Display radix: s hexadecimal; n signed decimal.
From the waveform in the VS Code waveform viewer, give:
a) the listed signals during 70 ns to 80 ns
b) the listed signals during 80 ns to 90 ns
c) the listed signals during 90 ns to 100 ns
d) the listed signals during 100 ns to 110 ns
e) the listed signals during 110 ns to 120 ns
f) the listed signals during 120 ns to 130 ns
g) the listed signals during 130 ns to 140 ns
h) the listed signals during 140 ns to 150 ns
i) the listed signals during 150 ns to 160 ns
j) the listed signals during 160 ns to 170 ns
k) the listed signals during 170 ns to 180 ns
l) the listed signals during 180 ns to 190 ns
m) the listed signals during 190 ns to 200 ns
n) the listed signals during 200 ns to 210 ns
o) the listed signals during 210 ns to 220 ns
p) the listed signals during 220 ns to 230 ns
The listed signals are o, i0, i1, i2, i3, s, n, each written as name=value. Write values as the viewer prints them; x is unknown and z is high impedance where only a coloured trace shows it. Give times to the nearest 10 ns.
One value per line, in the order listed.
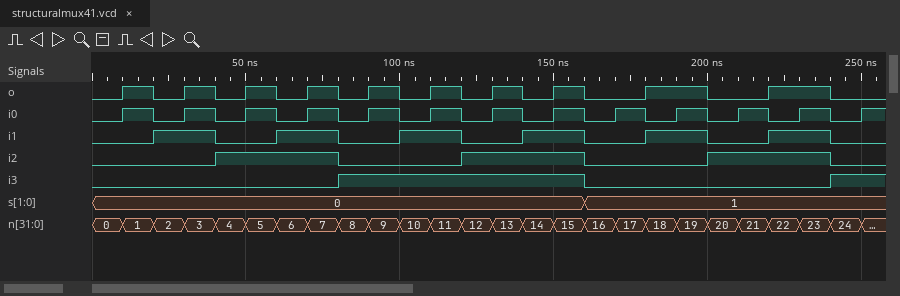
o=1, i0=1, i1=1, i2=1, i3=0, s=0, n=7
o=0, i0=0, i1=0, i2=0, i3=1, s=0, n=8
o=1, i0=1, i1=0, i2=0, i3=1, s=0, n=9
o=0, i0=0, i1=1, i2=0, i3=1, s=0, n=10
o=1, i0=1, i1=1, i2=0, i3=1, s=0, n=11
o=0, i0=0, i1=0, i2=1, i3=1, s=0, n=12
o=1, i0=1, i1=0, i2=1, i3=1, s=0, n=13
o=0, i0=0, i1=1, i2=1, i3=1, s=0, n=14
o=1, i0=1, i1=1, i2=1, i3=1, s=0, n=15
o=0, i0=0, i1=0, i2=0, i3=0, s=1, n=16
o=0, i0=1, i1=0, i2=0, i3=0, s=1, n=17
o=1, i0=0, i1=1, i2=0, i3=0, s=1, n=18
o=1, i0=1, i1=1, i2=0, i3=0, s=1, n=19
o=0, i0=0, i1=0, i2=1, i3=0, s=1, n=20
o=0, i0=1, i1=0, i2=1, i3=0, s=1, n=21
o=1, i0=0, i1=1, i2=1, i3=0, s=1, n=22
